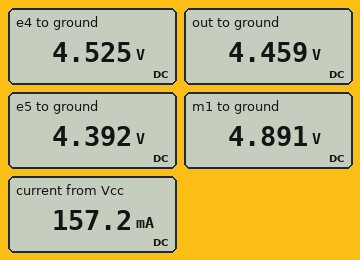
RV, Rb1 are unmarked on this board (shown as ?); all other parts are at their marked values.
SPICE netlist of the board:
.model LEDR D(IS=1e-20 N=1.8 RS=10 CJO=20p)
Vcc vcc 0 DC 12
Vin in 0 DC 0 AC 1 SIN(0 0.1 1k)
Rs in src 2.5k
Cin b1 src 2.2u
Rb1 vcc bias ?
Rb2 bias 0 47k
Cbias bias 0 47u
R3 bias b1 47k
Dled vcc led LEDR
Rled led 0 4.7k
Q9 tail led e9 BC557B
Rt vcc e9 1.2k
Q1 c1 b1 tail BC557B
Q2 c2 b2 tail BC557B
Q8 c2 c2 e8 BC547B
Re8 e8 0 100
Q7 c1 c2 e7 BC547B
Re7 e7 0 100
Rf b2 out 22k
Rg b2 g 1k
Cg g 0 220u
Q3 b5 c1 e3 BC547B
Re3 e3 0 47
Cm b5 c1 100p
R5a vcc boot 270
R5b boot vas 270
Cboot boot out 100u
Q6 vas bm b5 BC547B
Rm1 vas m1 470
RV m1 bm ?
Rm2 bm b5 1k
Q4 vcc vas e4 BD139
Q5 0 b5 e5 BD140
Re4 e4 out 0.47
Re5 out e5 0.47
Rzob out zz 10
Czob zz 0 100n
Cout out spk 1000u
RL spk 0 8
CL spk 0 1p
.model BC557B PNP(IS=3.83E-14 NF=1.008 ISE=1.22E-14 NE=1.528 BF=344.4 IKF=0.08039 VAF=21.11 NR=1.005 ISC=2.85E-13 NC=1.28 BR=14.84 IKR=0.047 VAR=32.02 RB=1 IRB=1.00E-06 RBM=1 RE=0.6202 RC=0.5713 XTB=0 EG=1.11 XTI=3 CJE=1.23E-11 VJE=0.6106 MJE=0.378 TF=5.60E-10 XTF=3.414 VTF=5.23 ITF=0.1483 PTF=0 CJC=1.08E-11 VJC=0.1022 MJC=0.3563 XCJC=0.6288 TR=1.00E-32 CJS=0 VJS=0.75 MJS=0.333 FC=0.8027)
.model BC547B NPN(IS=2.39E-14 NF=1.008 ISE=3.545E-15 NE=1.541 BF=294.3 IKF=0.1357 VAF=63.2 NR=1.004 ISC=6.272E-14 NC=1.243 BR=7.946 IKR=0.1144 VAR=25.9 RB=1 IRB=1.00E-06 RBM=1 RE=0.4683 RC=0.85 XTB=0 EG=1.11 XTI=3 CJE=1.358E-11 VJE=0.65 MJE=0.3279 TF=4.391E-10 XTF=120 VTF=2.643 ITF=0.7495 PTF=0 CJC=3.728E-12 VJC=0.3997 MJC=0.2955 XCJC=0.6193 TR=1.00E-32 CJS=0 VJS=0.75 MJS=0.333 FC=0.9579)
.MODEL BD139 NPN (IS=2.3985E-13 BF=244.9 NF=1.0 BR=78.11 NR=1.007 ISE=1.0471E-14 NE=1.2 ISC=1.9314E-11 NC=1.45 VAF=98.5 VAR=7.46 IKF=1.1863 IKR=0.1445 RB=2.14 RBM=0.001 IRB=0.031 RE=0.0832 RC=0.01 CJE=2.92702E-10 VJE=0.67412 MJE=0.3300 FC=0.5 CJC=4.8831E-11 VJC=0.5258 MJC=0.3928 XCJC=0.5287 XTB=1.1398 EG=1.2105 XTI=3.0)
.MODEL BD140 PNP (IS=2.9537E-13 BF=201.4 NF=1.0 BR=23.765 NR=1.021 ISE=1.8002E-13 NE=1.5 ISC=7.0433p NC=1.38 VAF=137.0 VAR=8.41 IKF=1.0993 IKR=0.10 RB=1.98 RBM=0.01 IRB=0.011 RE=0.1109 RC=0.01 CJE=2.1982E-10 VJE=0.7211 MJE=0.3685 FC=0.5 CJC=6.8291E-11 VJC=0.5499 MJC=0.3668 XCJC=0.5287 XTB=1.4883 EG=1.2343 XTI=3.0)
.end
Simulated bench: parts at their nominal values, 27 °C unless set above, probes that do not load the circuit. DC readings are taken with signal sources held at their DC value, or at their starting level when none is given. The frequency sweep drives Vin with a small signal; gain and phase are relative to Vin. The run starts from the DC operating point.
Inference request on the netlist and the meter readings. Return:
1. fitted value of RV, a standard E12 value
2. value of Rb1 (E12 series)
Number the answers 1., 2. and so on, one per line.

1. 680 Ω
2. 82 kΩ
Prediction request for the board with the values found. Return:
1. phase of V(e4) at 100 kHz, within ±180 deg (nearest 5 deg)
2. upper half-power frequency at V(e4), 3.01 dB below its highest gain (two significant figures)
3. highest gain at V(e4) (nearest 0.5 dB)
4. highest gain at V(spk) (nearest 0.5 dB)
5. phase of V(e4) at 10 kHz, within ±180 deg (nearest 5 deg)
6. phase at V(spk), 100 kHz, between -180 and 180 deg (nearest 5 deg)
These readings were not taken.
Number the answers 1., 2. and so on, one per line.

1. -5 deg
2. 1.4 MHz
3. 27.0 dB
4. 27.0 dB
5. 0 deg
6. -5 deg
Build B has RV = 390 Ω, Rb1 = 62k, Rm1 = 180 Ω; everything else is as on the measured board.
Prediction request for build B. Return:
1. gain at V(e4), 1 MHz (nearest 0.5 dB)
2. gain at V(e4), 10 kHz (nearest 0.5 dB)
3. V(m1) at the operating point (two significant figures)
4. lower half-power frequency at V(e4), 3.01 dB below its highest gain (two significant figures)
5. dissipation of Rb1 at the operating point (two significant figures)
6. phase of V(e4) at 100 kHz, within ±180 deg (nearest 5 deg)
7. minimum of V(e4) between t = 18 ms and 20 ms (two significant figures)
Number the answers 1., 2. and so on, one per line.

1. 12.5 dB
2. 26.5 dB
3. 5.7 V
4. 1.9 Hz
5. 740 µW
6. -20 deg
7. 3.1 V
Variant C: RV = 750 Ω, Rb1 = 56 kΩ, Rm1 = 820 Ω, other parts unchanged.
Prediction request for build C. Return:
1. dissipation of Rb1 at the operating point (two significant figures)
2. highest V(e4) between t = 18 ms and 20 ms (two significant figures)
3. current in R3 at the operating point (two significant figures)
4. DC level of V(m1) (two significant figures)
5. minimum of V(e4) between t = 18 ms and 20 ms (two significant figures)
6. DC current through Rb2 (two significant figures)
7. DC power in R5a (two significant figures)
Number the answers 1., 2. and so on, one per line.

1. 750 µW
2. 7.9 V
3. 1.4 µA
4. 5.9 V
5. 3.5 V
6. 120 µA
7. 28 mW
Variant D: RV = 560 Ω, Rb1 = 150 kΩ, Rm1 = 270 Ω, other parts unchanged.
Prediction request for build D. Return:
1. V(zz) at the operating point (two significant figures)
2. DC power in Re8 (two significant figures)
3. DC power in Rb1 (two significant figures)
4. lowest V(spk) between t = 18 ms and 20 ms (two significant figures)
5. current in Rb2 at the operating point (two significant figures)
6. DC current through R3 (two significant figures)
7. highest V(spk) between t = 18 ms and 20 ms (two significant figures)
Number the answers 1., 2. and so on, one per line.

1. 3.0 V
2. 24 µW
3. 550 µW
4. -1.4 V
5. 62 µA
6. 1.6 µA
7. 2.0 V
